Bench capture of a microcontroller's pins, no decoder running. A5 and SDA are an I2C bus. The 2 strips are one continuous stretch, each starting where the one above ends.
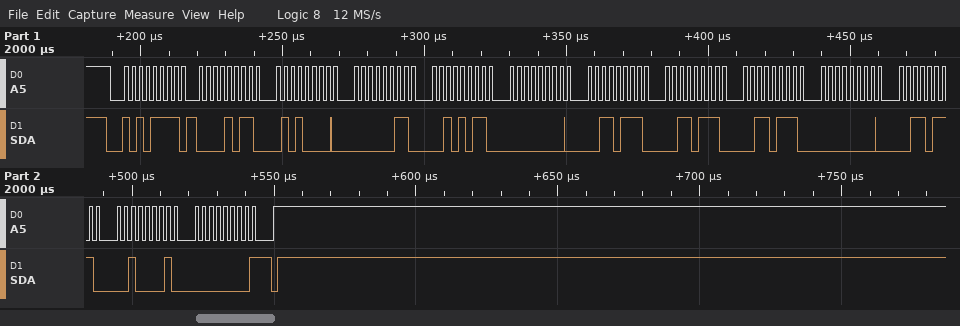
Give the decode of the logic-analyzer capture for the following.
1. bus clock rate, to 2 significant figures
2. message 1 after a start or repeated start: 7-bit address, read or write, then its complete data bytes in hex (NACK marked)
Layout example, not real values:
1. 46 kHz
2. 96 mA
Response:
1. 400 kHz
2. 0x57 read: 0B 50 03 2B 00 37 37 37 00 37 21 00 NACK
